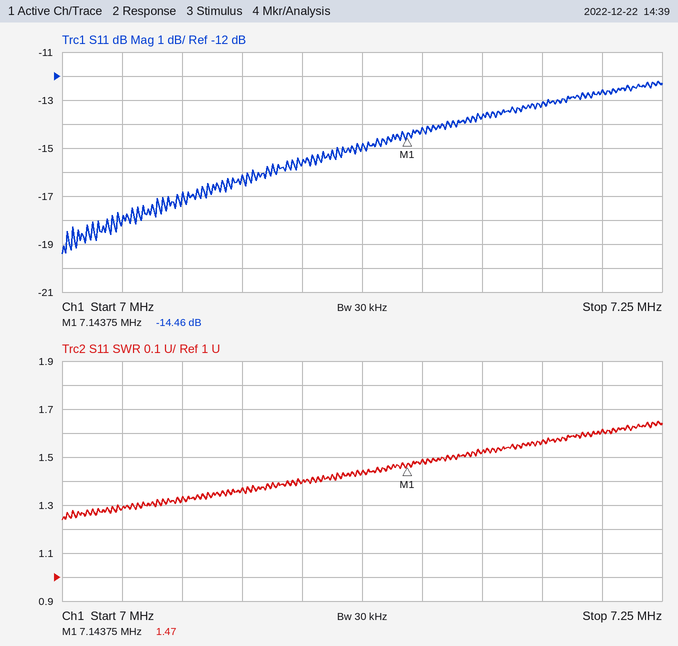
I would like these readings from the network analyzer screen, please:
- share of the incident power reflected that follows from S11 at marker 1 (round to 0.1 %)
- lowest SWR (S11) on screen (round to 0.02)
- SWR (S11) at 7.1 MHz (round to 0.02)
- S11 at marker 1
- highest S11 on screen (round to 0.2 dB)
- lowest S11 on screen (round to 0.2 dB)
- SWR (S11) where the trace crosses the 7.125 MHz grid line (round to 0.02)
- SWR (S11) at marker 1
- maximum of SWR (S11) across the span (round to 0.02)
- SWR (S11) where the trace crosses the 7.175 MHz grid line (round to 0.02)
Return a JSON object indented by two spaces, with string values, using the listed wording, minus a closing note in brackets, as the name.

{
  "share of the incident power reflected that follows from S11 at marker 1": "3.6 %",
  "lowest SWR (S11) on screen": "1.24",
  "SWR (S11) at 7.1 MHz": "1.40",
  "S11 at marker 1": "-14.46 dB",
  "highest S11 on screen": "-12.2 dB",
  "lowest S11 on screen": "-19.4 dB",
  "SWR (S11) where the trace crosses the 7.125 MHz grid line": "1.44",
  "SWR (S11) at marker 1": "1.47",
  "maximum of SWR (S11) across the span": "1.64",
  "SWR (S11) where the trace crosses the 7.175 MHz grid line": "1.52"
}
